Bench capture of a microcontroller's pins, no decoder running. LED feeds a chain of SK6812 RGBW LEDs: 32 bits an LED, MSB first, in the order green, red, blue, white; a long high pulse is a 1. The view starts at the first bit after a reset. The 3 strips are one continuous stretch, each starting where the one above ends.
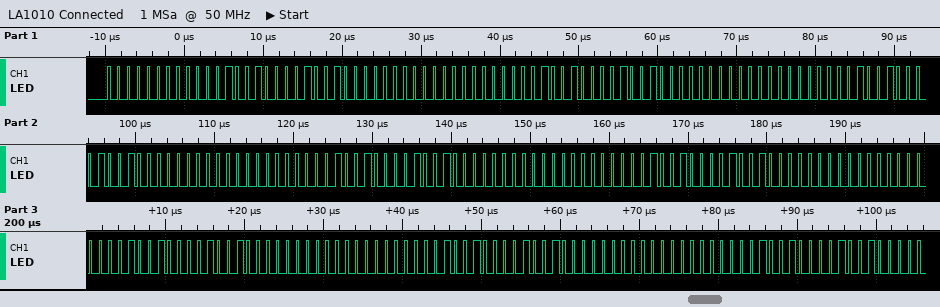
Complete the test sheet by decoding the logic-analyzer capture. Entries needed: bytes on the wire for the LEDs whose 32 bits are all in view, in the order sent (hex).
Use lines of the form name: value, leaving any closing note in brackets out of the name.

bytes on the wire for the LEDs whose 32 bits are all in view, in the order sent: 00 09 09 00 00 09 09 00 00 09 09 00 00 09 09 00 00 09 09 00 00 09 09 00 00 09 09 00
